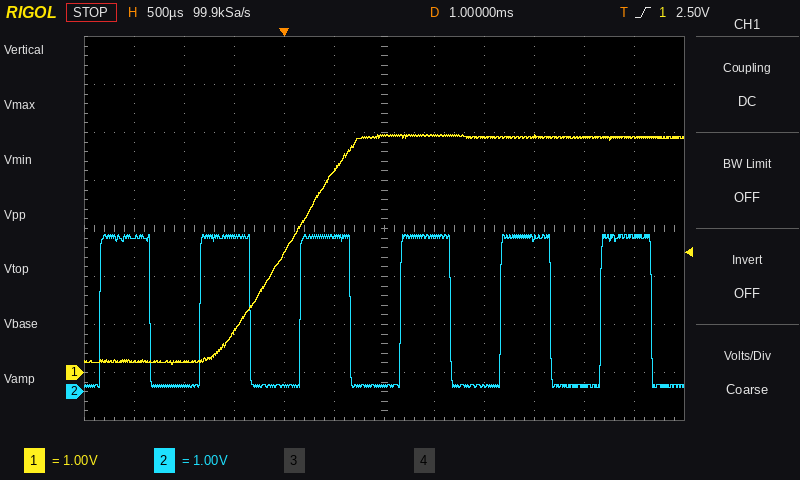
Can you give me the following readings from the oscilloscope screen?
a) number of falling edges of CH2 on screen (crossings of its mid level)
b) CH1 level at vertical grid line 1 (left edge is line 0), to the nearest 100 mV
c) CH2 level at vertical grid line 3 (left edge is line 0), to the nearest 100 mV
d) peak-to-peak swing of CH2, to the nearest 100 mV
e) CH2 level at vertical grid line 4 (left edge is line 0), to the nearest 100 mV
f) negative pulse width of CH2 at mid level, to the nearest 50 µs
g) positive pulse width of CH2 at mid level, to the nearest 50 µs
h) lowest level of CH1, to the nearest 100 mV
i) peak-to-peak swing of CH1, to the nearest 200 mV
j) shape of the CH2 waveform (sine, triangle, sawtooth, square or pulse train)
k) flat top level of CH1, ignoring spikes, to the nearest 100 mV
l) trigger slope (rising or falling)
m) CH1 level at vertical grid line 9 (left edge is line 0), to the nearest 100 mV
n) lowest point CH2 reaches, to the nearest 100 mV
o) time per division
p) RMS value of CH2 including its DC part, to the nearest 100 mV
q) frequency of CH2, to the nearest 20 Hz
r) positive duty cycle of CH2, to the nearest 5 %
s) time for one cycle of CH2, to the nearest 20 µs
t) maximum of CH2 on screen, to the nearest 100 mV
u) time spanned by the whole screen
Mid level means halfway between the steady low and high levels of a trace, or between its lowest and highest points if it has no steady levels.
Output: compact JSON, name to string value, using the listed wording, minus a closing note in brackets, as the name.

{"number of falling edges of CH2 on screen": "6", "CH1 level at vertical grid line 1 (left edge is line 0), to the nearest 100 mV": "200 mV", "CH2 level at vertical grid line 3 (left edge is line 0), to the nearest 100 mV": "3.2 V", "peak-to-peak swing of CH2, to the nearest 100 mV": "3.2 V", "CH2 level at vertical grid line 4 (left edge is line 0), to the nearest 100 mV": "100 mV", "negative pulse width of CH2 at mid level, to the nearest 50 µs": "500 µs", "positive pulse width of CH2 at mid level, to the nearest 50 µs": "500 µs", "lowest level of CH1, to the nearest 100 mV": "200 mV", "peak-to-peak swing of CH1, to the nearest 200 mV": "4.8 V", "shape of the CH2 waveform": "square", "flat top level of CH1, ignoring spikes, to the nearest 100 mV": "4.9 V", "trigger slope": "rising", "CH1 level at vertical grid line 9 (left edge is line 0), to the nearest 100 mV": "4.9 V", "lowest point CH2 reaches, to the nearest 100 mV": "100 mV", "time per division": "500 µs", "RMS value of CH2 including its DC part, to the nearest 100 mV": "2.3 V", "frequency of CH2, to the nearest 20 Hz": "1.00 kHz", "positive duty cycle of CH2, to the nearest 5 %": "50 %", "time for one cycle of CH2, to the nearest 20 µs": "1.00 ms", "maximum of CH2 on screen, to the nearest 100 mV": "3.3 V", "time spanned by the whole screen": "6 ms"}
